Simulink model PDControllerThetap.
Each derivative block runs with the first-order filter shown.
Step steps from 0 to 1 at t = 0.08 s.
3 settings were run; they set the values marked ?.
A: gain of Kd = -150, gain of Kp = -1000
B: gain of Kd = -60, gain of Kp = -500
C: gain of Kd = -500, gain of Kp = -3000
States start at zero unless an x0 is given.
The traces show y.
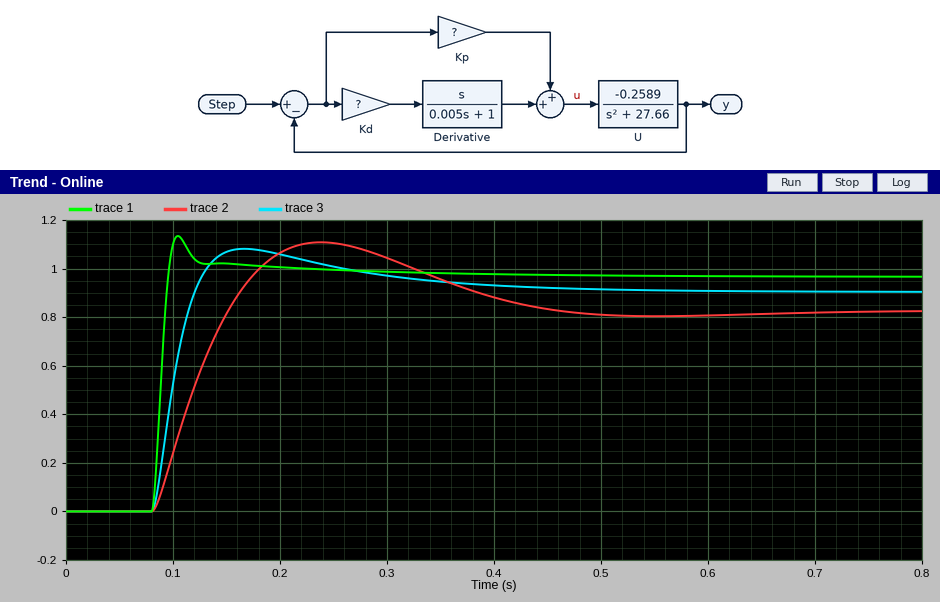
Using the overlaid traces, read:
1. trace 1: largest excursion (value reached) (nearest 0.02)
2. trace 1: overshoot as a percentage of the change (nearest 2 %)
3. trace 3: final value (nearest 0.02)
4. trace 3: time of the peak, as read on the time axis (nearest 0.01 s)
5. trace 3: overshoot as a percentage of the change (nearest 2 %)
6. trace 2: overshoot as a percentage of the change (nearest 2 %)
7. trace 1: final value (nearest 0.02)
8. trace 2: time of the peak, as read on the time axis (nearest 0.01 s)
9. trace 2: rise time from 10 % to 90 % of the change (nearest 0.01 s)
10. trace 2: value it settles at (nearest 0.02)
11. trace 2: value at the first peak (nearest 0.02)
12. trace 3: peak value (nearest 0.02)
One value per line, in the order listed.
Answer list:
1.14
18 %
0.90
0.17 s
20 %
34 %
0.96
0.24 s
0.05 s
0.82
1.10
1.08
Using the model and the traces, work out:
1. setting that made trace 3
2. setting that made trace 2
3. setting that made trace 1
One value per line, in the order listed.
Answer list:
A
B
C
